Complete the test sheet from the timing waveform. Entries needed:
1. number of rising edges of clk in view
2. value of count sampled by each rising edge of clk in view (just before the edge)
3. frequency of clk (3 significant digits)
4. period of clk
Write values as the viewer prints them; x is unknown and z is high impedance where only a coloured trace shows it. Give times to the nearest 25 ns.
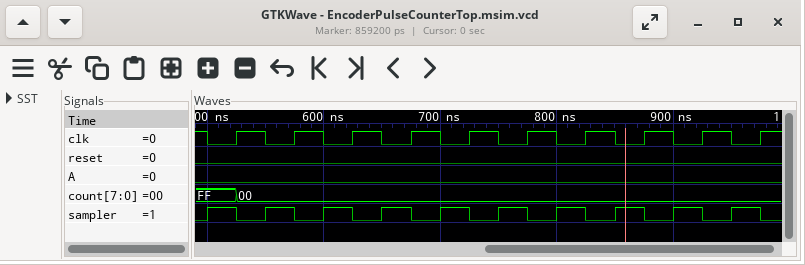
10
FF, 00, 00, 00, 00, 00, 00, 00, 00, 00
20.0 MHz
50 ns
